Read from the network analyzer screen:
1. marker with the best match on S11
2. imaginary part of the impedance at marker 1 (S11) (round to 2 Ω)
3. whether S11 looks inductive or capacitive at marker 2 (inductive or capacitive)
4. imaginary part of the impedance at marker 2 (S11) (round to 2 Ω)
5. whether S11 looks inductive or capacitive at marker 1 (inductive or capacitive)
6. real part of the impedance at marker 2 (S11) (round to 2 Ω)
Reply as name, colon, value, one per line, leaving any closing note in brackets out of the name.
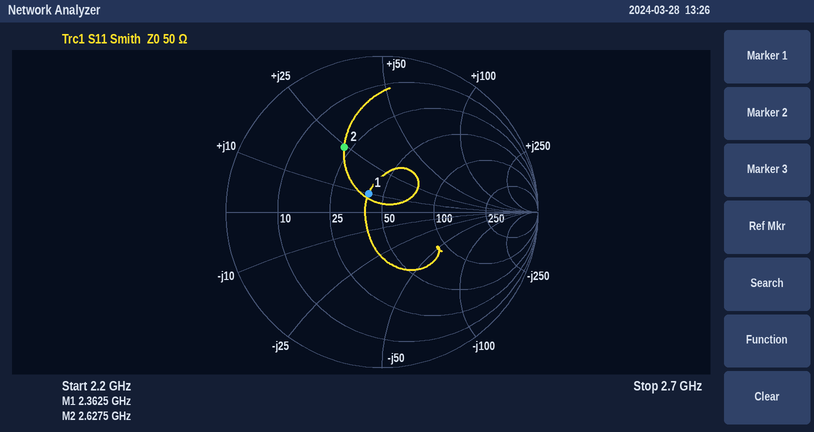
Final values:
marker with the best match on S11: marker 1
imaginary part of the impedance at marker 1 (S11): +10 Ω
whether S11 looks inductive or capacitive at marker 2: inductive
imaginary part of the impedance at marker 2 (S11): +24 Ω
whether S11 looks inductive or capacitive at marker 1: inductive
real part of the impedance at marker 2 (S11): 22 Ω
